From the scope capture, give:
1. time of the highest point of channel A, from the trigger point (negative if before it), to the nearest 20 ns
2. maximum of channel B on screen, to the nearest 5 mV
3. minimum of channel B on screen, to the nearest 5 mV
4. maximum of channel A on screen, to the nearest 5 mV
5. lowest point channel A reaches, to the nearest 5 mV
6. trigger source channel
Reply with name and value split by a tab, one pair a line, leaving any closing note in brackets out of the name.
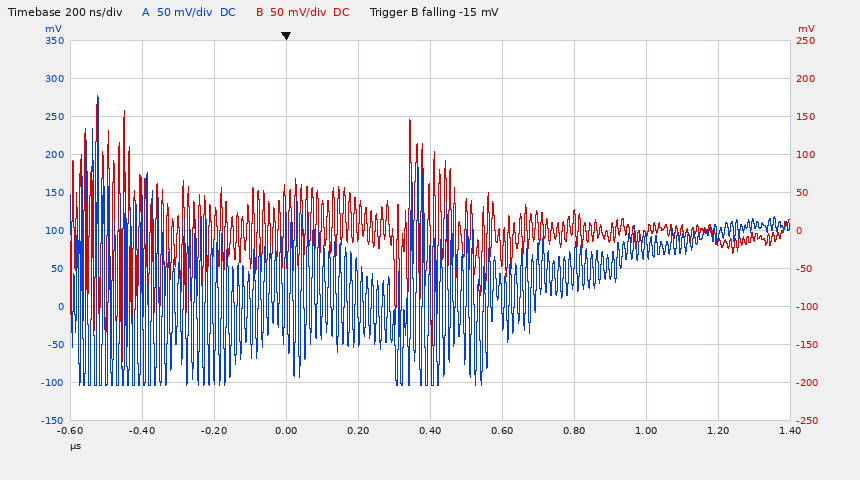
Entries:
time of the highest point of channel A, from the trigger point (negative if before it), to the nearest 20 ns	-520 ns
maximum of channel B on screen, to the nearest 5 mV	165 mV
minimum of channel B on screen, to the nearest 5 mV	-180 mV
maximum of channel A on screen, to the nearest 5 mV	280 mV
lowest point channel A reaches, to the nearest 5 mV	-105 mV
trigger source channel	channel B
